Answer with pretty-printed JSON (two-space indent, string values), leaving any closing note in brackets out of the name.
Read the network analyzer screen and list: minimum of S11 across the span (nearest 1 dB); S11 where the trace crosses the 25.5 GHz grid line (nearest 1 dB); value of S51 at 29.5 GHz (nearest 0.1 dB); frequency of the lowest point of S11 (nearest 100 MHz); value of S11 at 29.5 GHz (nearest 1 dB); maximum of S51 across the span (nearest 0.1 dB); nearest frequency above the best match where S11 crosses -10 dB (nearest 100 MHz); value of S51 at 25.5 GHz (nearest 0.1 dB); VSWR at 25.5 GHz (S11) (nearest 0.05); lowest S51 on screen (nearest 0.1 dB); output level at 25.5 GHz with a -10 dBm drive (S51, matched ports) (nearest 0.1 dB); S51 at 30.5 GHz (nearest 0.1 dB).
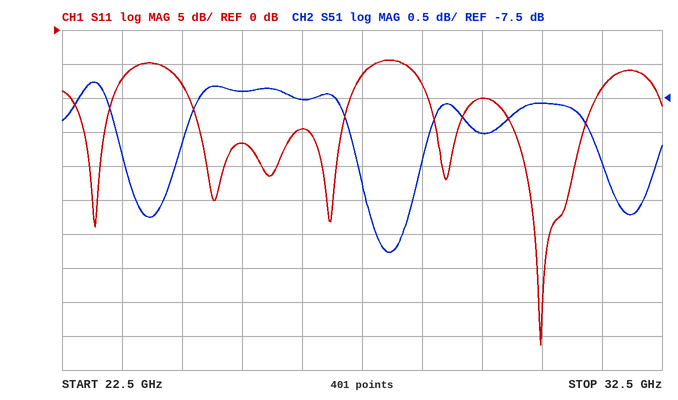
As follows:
{
  "minimum of S11 across the span": "-46 dB",
  "S11 where the trace crosses the 25.5 GHz grid line": "-17 dB",
  "value of S51 at 29.5 GHz": "-8.0 dB",
  "frequency of the lowest point of S11": "30.5 GHz",
  "value of S11 at 29.5 GHz": "-10 dB",
  "maximum of S51 across the span": "-7.3 dB",
  "nearest frequency above the best match where S11 crosses -10 dB": "31.4 GHz",
  "value of S51 at 25.5 GHz": "-7.4 dB",
  "VSWR at 25.5 GHz (S11)": "1.35",
  "lowest S51 on screen": "-9.8 dB",
  "output level at 25.5 GHz with a -10 dBm drive (S51, matched ports)": "-17.4 dBm",
  "S51 at 30.5 GHz": "-7.6 dB"
}
